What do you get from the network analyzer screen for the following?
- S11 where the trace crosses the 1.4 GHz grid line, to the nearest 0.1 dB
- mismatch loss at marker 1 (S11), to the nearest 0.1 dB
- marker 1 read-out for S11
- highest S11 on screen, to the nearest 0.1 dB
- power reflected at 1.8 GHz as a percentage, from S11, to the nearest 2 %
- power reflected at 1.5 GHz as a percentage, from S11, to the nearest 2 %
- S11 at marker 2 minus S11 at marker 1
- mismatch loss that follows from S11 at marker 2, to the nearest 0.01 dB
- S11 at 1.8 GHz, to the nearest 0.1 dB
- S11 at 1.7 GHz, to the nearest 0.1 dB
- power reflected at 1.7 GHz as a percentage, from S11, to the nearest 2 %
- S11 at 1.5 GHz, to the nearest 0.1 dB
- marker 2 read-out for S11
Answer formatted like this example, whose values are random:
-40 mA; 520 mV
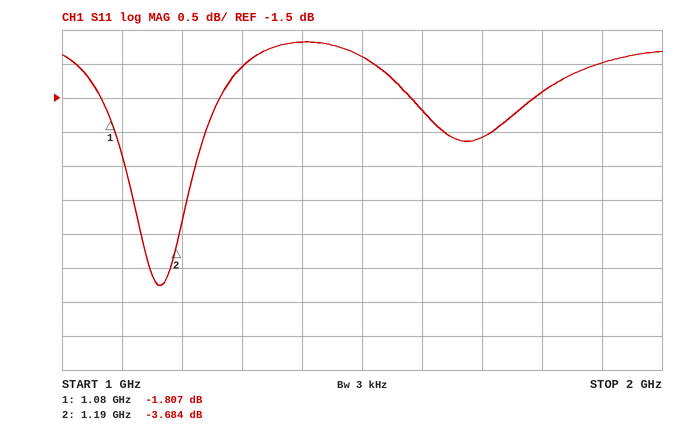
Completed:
-0.7 dB; 4.7 dB; -1.807 dB; -0.7 dB; 72 %; 82 %; -1.877 dB; 2.43 dB; -1.4 dB; -2.1 dB; 62 %; -0.9 dB; -3.684 dB
